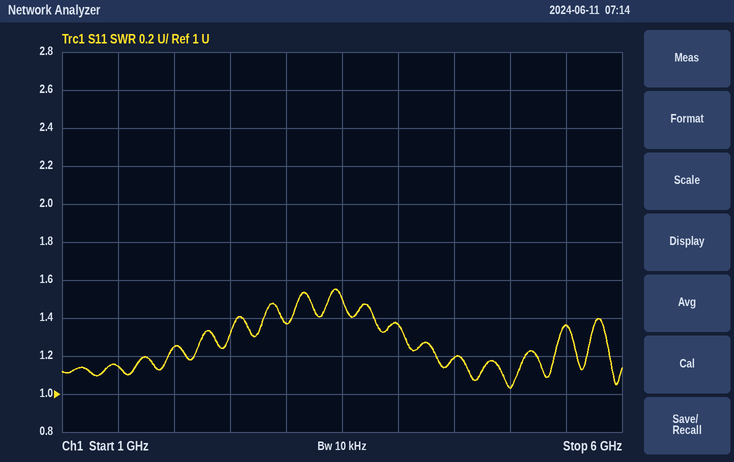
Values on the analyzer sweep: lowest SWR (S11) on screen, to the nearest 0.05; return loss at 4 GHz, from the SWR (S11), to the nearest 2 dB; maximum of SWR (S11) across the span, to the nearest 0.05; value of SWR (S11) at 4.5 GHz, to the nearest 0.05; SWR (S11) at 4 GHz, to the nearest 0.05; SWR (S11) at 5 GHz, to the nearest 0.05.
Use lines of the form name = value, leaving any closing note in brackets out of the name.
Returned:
lowest SWR (S11) on screen, to the nearest 0.05 = 1.05
return loss at 4 GHz, from the SWR (S11), to the nearest 2 dB = 16 dB
maximum of SWR (S11) across the span, to the nearest 0.05 = 1.55
value of SWR (S11) at 4.5 GHz, to the nearest 0.05 = 1.20
SWR (S11) at 4 GHz, to the nearest 0.05 = 1.35
SWR (S11) at 5 GHz, to the nearest 0.05 = 1.05
